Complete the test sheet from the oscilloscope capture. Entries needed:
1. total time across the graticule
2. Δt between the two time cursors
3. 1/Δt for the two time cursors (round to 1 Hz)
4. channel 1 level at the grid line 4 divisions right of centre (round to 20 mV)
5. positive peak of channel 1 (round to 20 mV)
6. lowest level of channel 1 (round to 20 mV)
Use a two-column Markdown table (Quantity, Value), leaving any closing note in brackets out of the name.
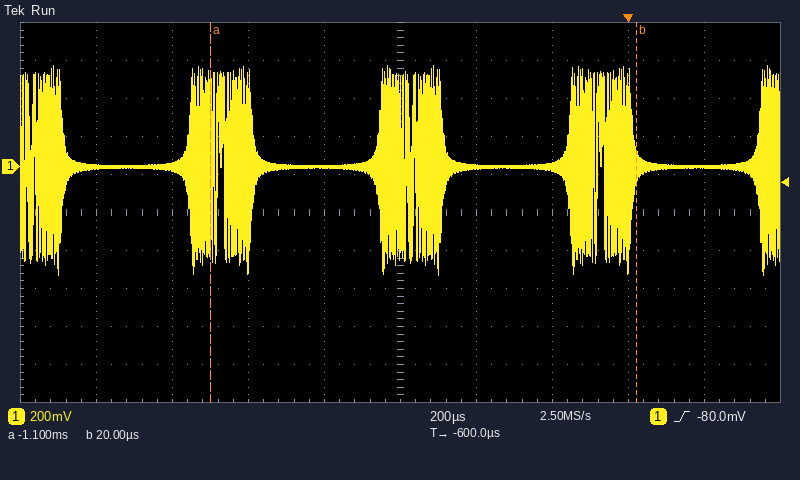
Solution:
| Quantity | Value |
|---|---|
| total time across the graticule | 2 ms |
| Δt between the two time cursors | 1.12 ms |
| 1/Δt for the two time cursors | 893 Hz |
| channel 1 level at the grid line 4 divisions right of centre | 0 mV |
| positive peak of channel 1 | 540 mV |
| lowest level of channel 1 | -580 mV |
